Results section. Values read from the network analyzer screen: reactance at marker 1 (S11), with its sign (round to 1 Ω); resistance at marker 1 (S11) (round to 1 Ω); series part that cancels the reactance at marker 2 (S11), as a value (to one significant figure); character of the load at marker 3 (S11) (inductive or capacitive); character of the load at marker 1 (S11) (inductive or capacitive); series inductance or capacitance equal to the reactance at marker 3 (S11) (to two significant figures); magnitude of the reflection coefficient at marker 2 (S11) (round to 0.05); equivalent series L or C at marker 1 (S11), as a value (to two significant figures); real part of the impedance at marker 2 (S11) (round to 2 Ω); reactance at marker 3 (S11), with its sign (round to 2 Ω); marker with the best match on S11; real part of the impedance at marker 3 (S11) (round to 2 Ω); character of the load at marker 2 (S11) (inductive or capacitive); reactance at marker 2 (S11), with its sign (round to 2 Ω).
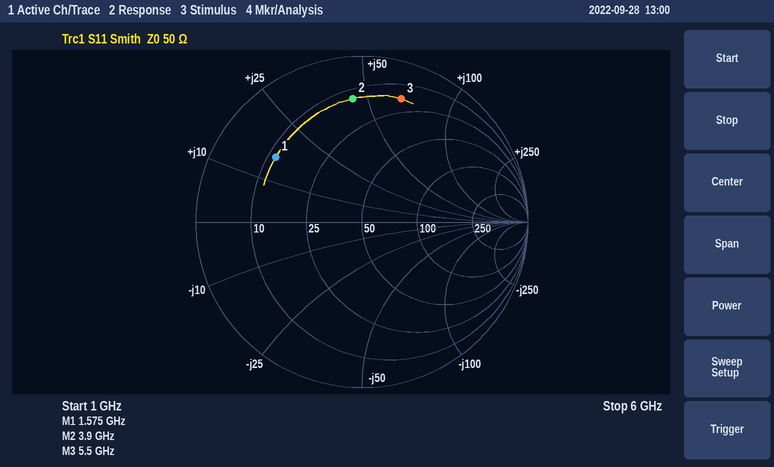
+16 Ω
12 Ω
900 fF
inductive
inductive
1.9 nH
0.75
1.6 nH
14 Ω
+66 Ω
marker 1
18 Ω
inductive
+44 Ω
